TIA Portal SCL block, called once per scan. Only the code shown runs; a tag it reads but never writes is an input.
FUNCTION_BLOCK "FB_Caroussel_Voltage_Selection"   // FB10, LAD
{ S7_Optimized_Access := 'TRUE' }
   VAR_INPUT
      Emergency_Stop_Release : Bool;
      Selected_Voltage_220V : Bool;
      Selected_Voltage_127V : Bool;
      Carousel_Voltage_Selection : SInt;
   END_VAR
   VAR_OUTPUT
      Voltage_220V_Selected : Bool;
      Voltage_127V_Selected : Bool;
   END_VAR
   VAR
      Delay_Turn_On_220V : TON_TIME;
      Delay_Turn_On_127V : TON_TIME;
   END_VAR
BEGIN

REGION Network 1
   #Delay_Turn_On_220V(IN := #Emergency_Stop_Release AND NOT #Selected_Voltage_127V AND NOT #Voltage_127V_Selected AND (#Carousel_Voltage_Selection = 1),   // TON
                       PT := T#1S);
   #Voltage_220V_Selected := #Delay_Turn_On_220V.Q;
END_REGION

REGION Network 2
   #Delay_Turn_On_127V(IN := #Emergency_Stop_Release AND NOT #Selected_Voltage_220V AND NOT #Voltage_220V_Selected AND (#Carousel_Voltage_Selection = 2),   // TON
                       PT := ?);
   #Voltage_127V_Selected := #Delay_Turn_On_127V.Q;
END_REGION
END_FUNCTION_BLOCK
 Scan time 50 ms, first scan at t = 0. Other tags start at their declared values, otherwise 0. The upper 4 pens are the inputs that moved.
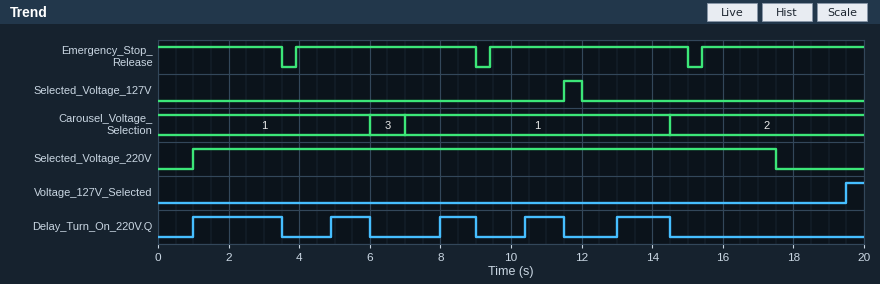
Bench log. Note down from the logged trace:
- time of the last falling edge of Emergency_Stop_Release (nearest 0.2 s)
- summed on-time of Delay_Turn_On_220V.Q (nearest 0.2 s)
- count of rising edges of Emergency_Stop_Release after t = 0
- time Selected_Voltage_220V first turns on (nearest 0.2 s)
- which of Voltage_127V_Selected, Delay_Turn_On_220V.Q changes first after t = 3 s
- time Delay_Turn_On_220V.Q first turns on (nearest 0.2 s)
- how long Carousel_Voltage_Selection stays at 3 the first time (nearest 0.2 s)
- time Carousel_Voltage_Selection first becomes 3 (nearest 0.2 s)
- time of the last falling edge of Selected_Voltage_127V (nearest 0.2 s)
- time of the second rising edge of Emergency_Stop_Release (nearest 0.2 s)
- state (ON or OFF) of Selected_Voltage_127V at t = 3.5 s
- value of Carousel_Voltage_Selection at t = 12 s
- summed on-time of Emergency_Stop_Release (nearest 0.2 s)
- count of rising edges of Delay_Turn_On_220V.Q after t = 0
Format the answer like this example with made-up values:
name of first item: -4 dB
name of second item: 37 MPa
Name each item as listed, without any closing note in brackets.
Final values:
time of the last falling edge of Emergency_Stop_Release: 15.0 s
summed on-time of Delay_Turn_On_220V.Q: 7.2 s
count of rising edges of Emergency_Stop_Release after t = 0: 3
time Selected_Voltage_220V first turns on: 1.0 s
which of Voltage_127V_Selected, Delay_Turn_On_220V.Q changes first after t = 3 s: Delay_Turn_On_220V.Q
time Delay_Turn_On_220V.Q first turns on: 1.0 s
how long Carousel_Voltage_Selection stays at 3 the first time: 1.0 s
time Carousel_Voltage_Selection first becomes 3: 6.0 s
time of the last falling edge of Selected_Voltage_127V: 12.0 s
time of the second rising edge of Emergency_Stop_Release: 9.4 s
state (ON or OFF) of Selected_Voltage_127V at t = 3.5 s: OFF
value of Carousel_Voltage_Selection at t = 12 s: 1
summed on-time of Emergency_Stop_Release: 18.8 s
count of rising edges of Delay_Turn_On_220V.Q after t = 0: 5
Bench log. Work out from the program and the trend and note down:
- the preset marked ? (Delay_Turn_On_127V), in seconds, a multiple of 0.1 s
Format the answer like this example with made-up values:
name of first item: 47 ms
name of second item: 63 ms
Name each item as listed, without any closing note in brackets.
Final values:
the preset marked ? (Delay_Turn_On_127V), in seconds, a multiple of 0.1 s: 2.0 s
